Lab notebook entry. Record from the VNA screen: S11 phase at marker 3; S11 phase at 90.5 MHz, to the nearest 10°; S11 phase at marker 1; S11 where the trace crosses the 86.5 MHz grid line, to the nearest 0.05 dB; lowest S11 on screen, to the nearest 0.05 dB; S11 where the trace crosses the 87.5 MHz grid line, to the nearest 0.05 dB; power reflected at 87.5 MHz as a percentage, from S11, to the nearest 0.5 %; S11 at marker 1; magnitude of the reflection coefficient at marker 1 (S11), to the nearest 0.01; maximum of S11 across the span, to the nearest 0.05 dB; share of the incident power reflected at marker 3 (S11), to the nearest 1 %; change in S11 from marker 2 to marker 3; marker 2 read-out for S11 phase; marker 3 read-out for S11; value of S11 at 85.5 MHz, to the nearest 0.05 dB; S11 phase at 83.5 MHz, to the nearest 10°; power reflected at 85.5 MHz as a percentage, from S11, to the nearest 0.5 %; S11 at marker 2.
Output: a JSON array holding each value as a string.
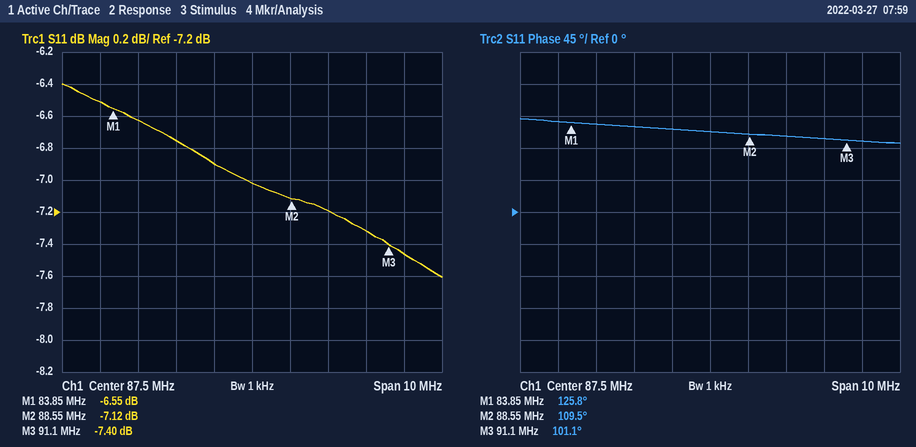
["101.1°", "100°", "125.8°", "-6.90 dB", "-7.60 dB", "-7.00 dB", "20.0 %", "-6.55 dB", "0.47", "-6.40 dB", "18 %", "-0.28 dB", "109.5°", "-7.40 dB", "-6.75 dB", "130°", "21.0 %", "-7.12 dB"]
